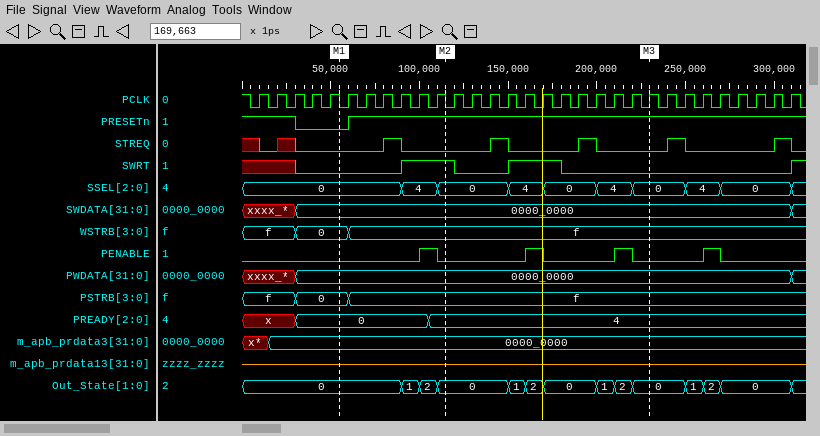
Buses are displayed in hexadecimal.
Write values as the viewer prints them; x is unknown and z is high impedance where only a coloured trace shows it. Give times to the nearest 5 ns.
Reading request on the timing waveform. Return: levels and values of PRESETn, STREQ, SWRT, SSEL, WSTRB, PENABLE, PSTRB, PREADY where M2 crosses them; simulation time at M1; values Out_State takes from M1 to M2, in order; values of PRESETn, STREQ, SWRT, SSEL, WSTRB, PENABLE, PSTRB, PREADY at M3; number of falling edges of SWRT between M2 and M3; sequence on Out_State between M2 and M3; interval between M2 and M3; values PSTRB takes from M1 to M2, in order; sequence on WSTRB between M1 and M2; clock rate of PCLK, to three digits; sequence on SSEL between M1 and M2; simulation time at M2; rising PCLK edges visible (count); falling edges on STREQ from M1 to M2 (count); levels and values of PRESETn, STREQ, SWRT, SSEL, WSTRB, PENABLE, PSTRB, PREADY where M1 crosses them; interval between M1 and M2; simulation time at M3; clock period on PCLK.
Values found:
PRESETn=1, STREQ=0, SWRT=1, SSEL=0, WSTRB=f, PENABLE=0, PSTRB=f, PREADY=4
55 ns
0, 1, 2, 0
PRESETn=1, STREQ=0, SWRT=0, SSEL=0, WSTRB=f, PENABLE=0, PSTRB=f, PREADY=4
2
0, 1, 2, 0, 1, 2, 0
115 ns
0, f
0, f
100 MHz
0, 4, 0
115 ns
31
1
PRESETn=0, STREQ=0, SWRT=0, SSEL=0, WSTRB=0, PENABLE=0, PSTRB=0, PREADY=0
60 ns
230 ns
10 ns
